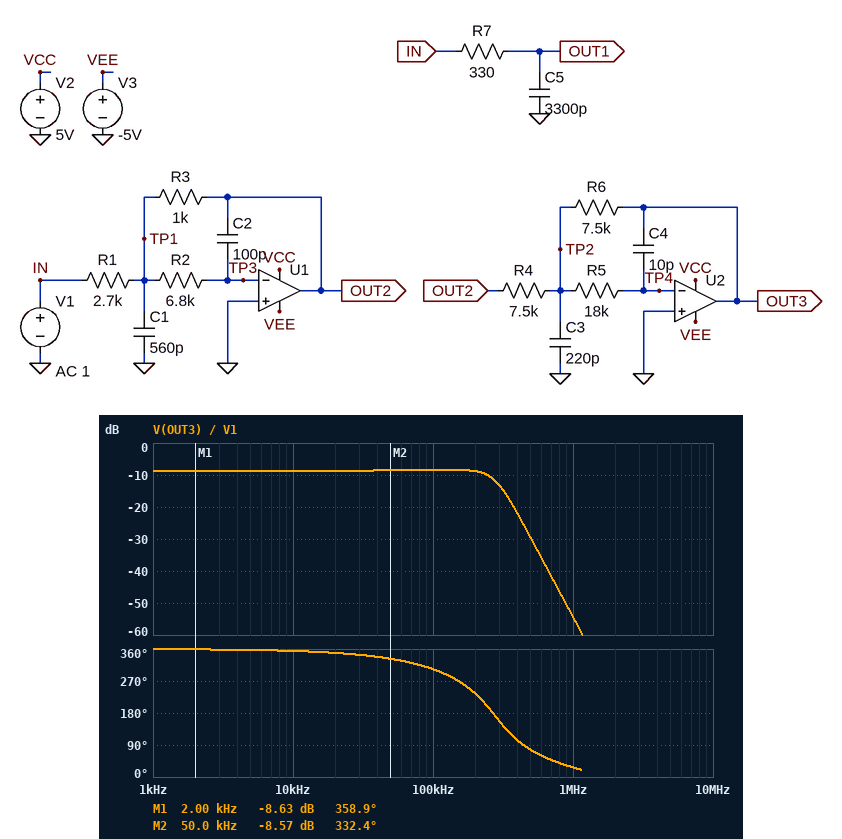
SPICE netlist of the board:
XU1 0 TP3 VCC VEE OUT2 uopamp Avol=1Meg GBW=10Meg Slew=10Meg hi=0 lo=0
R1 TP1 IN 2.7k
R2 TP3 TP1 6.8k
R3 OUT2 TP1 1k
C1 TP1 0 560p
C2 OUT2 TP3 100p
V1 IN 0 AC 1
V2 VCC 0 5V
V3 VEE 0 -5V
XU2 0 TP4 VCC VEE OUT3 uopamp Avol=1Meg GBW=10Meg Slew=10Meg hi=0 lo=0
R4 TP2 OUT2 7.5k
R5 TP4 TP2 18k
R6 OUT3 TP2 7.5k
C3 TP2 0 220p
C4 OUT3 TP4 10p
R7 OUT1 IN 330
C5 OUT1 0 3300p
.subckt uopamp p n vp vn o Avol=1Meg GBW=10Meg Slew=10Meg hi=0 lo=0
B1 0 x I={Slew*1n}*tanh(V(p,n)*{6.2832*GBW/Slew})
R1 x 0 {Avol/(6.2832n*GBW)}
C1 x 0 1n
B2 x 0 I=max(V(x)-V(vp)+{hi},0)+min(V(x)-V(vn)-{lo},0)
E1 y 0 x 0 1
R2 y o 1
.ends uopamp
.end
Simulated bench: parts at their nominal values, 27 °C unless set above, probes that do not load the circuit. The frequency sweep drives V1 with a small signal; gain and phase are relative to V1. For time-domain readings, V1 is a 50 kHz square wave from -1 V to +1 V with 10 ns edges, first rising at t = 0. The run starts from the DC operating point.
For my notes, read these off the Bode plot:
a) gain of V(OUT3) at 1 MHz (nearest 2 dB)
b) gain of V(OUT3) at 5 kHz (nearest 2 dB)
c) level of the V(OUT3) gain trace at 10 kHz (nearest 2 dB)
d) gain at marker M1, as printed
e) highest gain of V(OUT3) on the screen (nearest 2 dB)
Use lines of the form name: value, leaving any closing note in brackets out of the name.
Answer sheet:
gain of V(OUT3) at 1 MHz: -54 dB
gain of V(OUT3) at 5 kHz: -8 dB
level of the V(OUT3) gain trace at 10 kHz: -8 dB
gain at marker M1, as printed: -8.63 dB
highest gain of V(OUT3) on the screen: -8 dB
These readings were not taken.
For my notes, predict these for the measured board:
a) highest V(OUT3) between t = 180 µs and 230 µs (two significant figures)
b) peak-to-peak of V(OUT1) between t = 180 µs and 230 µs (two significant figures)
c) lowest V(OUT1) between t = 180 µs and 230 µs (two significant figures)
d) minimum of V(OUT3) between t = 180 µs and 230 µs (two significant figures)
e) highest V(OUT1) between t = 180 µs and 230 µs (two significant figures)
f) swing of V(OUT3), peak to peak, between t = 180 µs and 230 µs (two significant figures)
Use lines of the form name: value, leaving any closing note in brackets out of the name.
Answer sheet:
highest V(OUT3) between t = 180 µs and 230 µs: 460 mV
peak-to-peak of V(OUT1) between t = 180 µs and 230 µs: 2.0 V
lowest V(OUT1) between t = 180 µs and 230 µs: -1.0 V
minimum of V(OUT3) between t = 180 µs and 230 µs: -460 mV
highest V(OUT1) between t = 180 µs and 230 µs: 1.0 V
swing of V(OUT3), peak to peak, between t = 180 µs and 230 µs: 930 mV
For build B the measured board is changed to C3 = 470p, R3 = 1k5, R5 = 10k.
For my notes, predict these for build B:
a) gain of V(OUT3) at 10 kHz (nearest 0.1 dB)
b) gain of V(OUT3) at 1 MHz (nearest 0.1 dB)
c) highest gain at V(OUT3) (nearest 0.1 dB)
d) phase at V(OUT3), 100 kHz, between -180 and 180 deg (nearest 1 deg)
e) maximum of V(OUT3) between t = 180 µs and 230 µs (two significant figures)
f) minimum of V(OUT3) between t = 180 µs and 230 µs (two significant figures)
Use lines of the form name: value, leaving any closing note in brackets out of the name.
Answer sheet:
gain of V(OUT3) at 10 kHz: -5.1 dB
gain of V(OUT3) at 1 MHz: -56.2 dB
highest gain at V(OUT3): -2.9 dB
phase at V(OUT3), 100 kHz, between -180 and 180 deg: -58 deg
maximum of V(OUT3) between t = 180 µs and 230 µs: 820 mV
minimum of V(OUT3) between t = 180 µs and 230 µs: -820 mV
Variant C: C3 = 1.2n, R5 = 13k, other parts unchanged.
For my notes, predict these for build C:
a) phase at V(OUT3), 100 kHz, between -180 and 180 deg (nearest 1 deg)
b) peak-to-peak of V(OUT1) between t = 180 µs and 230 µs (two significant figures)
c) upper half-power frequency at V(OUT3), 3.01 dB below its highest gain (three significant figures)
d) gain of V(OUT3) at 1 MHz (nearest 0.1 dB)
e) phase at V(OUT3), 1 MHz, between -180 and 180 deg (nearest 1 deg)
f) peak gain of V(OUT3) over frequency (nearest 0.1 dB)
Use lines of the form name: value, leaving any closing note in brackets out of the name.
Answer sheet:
phase at V(OUT3), 100 kHz, between -180 and 180 deg: -63 deg
peak-to-peak of V(OUT1) between t = 180 µs and 230 µs: 2.0 V
upper half-power frequency at V(OUT3), 3.01 dB below its highest gain: 154 kHz
gain of V(OUT3) at 1 MHz: -66.8 dB
phase at V(OUT3), 1 MHz, between -180 and 180 deg: 16 deg
peak gain of V(OUT3) over frequency: 0.6 dB
